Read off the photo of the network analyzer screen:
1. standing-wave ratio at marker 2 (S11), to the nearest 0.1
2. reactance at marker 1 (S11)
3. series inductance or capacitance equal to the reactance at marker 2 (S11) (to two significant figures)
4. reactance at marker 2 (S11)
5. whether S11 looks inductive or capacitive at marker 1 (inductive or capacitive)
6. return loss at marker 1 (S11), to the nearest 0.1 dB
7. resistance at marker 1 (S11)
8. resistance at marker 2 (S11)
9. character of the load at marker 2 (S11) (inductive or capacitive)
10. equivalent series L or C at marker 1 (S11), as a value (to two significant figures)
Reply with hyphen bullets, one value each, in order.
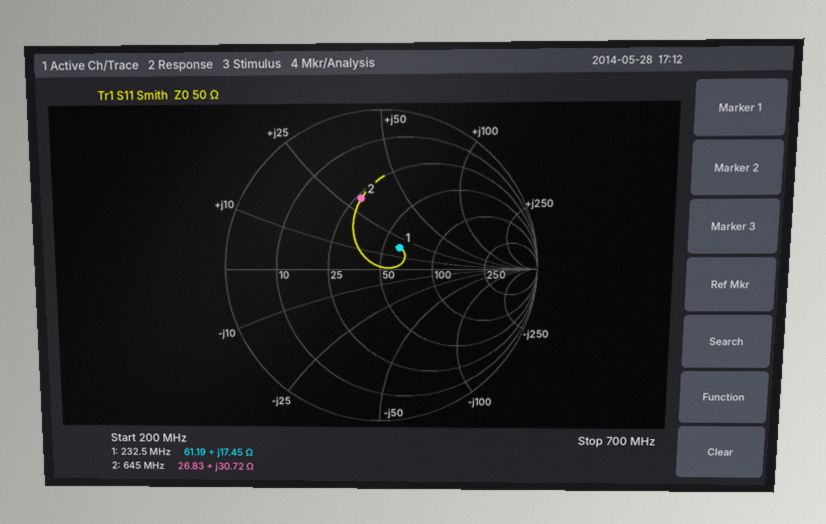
- 2.7
- +17.45 Ω
- 7.6 nH
- +30.72 Ω
- inductive
- 14.7 dB
- 61.19 Ω
- 26.83 Ω
- inductive
- 12 nH
